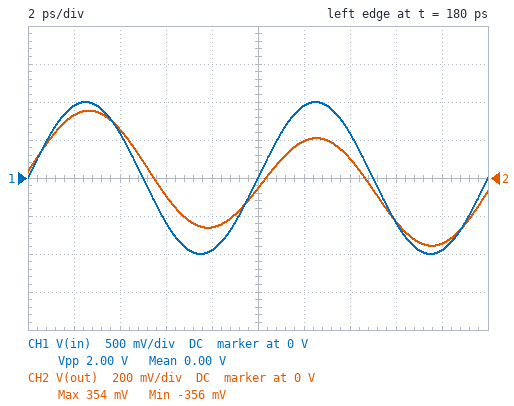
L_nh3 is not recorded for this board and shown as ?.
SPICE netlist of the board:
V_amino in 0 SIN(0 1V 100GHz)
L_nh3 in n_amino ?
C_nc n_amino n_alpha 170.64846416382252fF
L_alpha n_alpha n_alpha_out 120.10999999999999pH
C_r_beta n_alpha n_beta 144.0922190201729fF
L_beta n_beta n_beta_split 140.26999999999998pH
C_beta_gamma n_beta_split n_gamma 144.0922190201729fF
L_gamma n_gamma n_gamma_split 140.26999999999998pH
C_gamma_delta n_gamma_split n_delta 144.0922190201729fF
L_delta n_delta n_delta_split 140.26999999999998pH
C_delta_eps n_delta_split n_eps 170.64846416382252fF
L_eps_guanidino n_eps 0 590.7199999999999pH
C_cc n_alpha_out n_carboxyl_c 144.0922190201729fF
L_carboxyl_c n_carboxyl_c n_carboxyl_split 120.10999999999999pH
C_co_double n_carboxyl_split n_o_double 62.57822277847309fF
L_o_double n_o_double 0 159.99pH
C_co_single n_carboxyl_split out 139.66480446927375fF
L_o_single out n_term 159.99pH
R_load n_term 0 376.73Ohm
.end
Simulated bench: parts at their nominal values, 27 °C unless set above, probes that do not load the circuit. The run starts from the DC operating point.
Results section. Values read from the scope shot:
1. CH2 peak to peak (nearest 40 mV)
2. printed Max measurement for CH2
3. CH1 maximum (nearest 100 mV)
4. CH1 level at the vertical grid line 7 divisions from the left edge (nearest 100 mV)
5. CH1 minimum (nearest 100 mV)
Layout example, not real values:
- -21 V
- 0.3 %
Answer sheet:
- 720 mV
- 354 mV
- 1.0 V
- 600 mV
- -1.0 V
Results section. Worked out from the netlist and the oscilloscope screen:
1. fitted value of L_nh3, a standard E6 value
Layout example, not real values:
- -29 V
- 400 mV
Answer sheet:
- 68 pH
